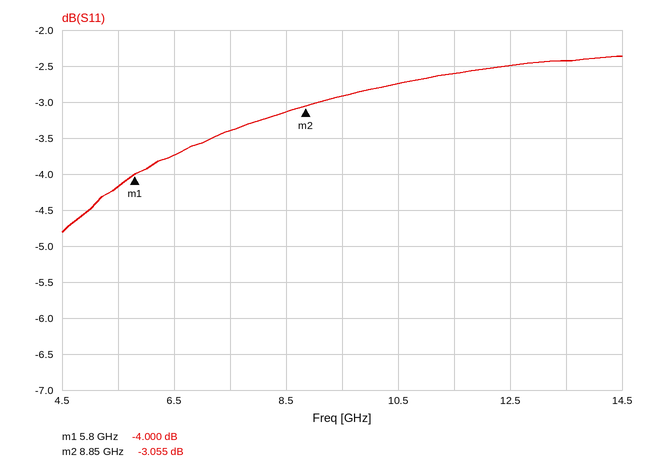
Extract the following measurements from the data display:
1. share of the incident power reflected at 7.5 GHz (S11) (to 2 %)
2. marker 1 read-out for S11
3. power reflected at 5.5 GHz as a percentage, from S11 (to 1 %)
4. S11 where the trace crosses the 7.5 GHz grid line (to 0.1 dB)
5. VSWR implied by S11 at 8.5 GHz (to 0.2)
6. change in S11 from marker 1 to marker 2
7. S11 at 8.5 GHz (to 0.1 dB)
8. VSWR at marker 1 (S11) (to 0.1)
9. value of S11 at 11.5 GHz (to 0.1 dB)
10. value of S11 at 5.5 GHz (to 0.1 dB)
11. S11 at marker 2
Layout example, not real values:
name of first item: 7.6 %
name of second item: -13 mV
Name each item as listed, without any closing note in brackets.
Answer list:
share of the incident power reflected at 7.5 GHz (S11): 46 %
marker 1 read-out for S11: -4.000 dB
power reflected at 5.5 GHz as a percentage, from S11: 38 %
S11 where the trace crosses the 7.5 GHz grid line: -3.4 dB
VSWR implied by S11 at 8.5 GHz: 5.6
change in S11 from marker 1 to marker 2: 0.945 dB
S11 at 8.5 GHz: -3.1 dB
VSWR at marker 1 (S11): 4.4
value of S11 at 11.5 GHz: -2.6 dB
value of S11 at 5.5 GHz: -4.2 dB
S11 at marker 2: -3.055 dB
